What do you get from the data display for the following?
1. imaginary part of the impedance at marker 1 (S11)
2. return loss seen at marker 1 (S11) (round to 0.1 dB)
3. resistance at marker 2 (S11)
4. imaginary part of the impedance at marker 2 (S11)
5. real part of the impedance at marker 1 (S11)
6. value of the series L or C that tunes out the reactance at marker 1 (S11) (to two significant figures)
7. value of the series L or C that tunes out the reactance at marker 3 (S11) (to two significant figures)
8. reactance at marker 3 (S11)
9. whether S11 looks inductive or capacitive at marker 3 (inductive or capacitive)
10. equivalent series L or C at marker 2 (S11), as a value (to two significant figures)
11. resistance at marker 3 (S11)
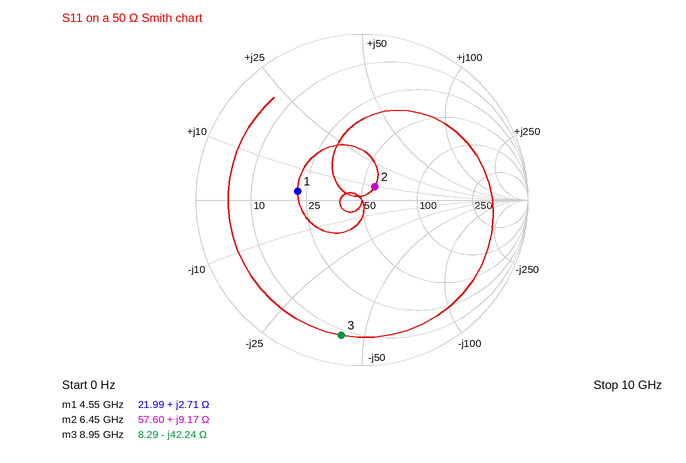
+2.71 Ω
8.2 dB
57.60 Ω
+9.17 Ω
21.99 Ω
13 pF
750 pH
-42.24 Ω
capacitive
230 pH
8.29 Ω
